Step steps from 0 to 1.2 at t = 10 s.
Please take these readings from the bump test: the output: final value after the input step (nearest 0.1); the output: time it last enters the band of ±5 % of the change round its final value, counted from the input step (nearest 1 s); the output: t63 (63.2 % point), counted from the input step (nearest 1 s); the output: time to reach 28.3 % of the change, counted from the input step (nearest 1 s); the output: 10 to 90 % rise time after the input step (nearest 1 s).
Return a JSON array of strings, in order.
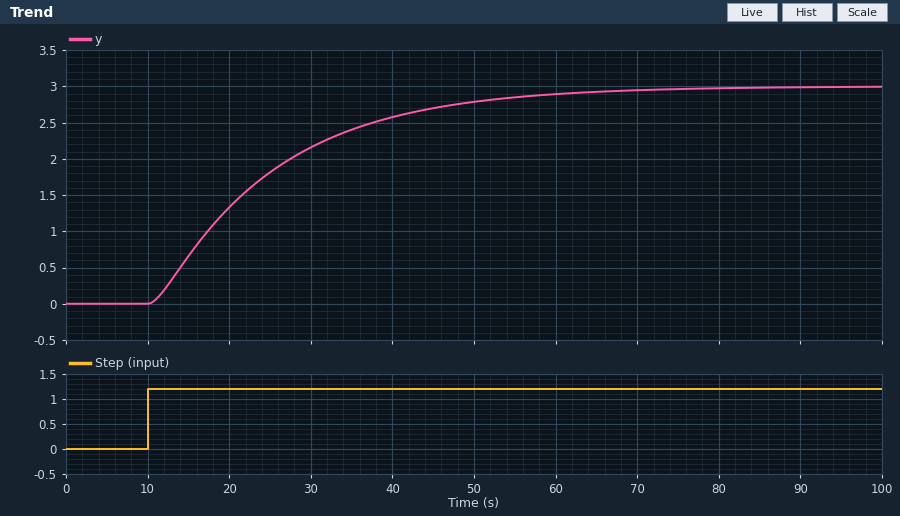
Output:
["3.0", "45 s", "16 s", "6 s", "32 s"]
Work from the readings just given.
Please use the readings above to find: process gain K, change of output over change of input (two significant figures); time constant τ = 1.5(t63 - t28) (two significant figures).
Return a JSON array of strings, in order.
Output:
["2.5", "15 s"]
